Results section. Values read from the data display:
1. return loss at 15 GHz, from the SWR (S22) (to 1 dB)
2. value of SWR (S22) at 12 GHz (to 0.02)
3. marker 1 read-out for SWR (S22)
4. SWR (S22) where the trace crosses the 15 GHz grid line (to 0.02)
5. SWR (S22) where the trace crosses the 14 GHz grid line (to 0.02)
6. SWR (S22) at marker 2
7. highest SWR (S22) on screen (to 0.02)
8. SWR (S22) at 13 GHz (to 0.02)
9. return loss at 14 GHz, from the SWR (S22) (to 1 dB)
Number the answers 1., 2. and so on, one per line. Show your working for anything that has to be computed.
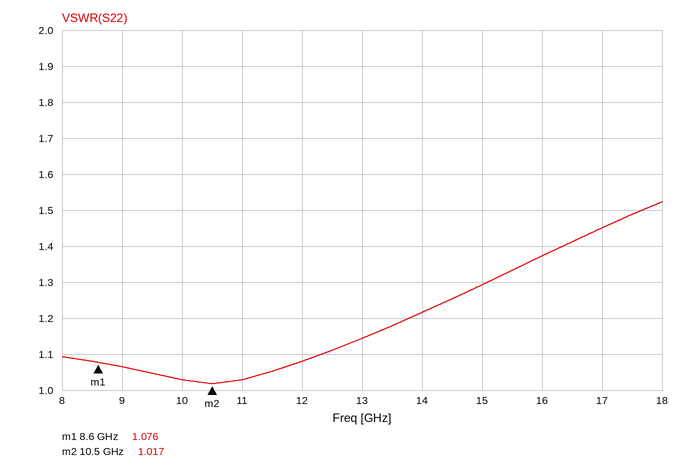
1. −20 log10((1.3 − 1)/(1.3 + 1)) ≈ 18 dB
2. 1.08
3. 1.076
4. 1.30
5. 1.22
6. 1.017
7. 1.52
8. 1.14
9. −20 log10((1.22 − 1)/(1.22 + 1)) ≈ 20 dB
